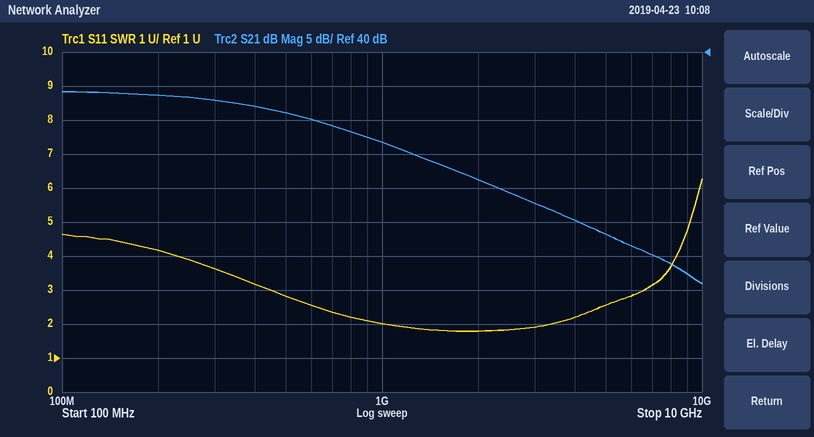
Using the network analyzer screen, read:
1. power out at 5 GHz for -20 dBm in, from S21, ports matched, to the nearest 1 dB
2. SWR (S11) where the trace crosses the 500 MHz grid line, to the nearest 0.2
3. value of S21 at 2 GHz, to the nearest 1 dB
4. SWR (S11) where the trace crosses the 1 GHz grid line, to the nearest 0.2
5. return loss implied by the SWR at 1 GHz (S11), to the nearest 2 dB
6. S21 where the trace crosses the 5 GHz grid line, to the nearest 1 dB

-7 dBm
2.8
21 dB
2.0
10 dB
13 dB
